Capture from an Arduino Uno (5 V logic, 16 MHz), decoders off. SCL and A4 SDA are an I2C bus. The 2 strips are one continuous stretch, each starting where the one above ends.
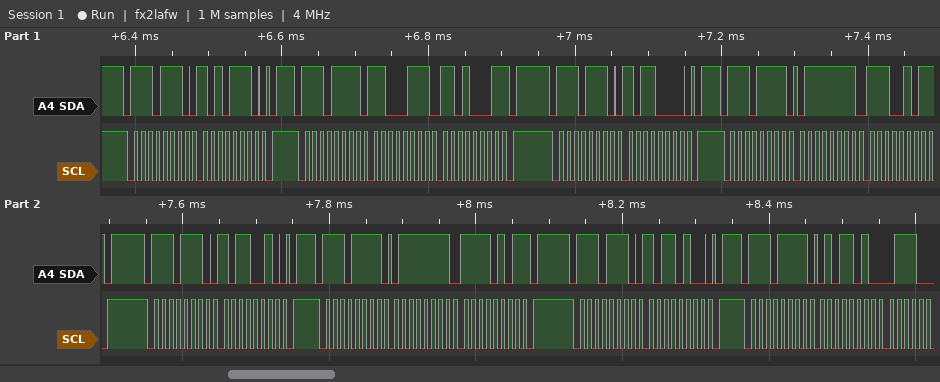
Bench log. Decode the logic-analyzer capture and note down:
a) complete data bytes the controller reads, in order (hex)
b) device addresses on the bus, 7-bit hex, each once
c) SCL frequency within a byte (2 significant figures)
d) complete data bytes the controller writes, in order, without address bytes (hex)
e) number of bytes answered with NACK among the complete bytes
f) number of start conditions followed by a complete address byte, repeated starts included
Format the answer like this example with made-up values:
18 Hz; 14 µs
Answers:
C7 D1 7F E5 7F F5 5A; 0x77; 100 kHz; AE B0 B2 B4; 3; 8
